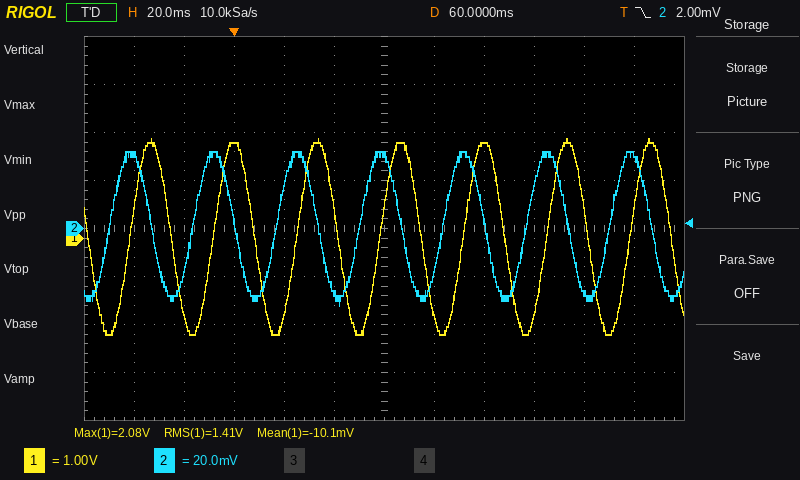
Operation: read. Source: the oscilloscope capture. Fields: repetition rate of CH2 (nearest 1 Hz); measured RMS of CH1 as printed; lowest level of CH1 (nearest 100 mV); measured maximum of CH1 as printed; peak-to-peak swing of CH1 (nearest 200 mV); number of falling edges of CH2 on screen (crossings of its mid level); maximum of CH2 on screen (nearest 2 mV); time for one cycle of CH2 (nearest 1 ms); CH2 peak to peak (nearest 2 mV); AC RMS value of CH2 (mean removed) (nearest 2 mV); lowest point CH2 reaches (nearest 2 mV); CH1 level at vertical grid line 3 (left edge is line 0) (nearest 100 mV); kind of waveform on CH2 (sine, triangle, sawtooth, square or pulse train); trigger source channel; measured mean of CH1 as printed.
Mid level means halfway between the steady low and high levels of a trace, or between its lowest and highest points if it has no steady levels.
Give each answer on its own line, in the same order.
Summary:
30 Hz
1.41 V
-2.0 V
2.08 V
4.0 V
7
32 mV
33 ms
64 mV
22 mV
-32 mV
2.0 V
sine
CH2
-10.1 mV
